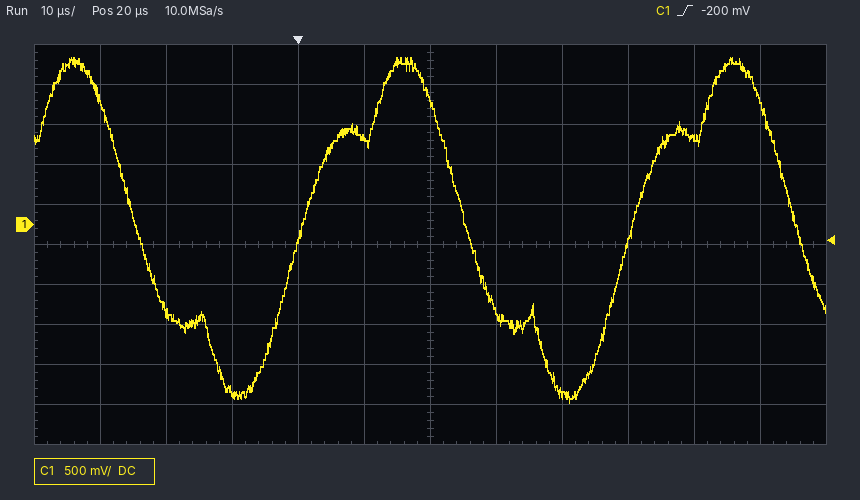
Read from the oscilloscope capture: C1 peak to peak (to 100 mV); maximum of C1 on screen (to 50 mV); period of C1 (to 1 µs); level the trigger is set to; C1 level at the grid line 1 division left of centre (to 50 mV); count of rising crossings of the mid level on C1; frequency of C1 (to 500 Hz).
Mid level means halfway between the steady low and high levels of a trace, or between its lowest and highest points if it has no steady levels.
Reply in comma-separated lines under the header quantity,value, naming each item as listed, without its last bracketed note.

quantity,value
C1 peak to peak,4.30 V
maximum of C1 on screen,2.10 V
period of C1,50 µs
level the trigger is set to,-200 mV
C1 level at the grid line 1 division left of centre,1.10 V
count of rising crossings of the mid level on C1,2
frequency of C1,20.0 kHz
